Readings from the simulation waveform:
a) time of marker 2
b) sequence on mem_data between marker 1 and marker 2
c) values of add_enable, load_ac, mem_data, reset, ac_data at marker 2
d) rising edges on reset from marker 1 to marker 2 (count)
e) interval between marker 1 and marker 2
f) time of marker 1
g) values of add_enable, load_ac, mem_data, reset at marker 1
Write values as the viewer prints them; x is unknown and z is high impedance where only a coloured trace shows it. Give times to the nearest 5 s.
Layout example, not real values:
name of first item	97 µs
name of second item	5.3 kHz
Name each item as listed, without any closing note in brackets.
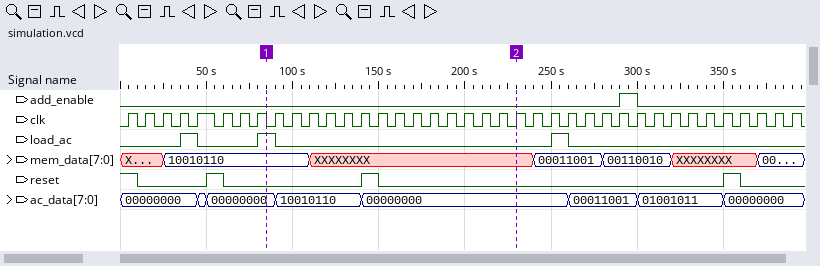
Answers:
time of marker 2	230 s
sequence on mem_data between marker 1 and marker 2	10010110, XXXXXXXX
values of add_enable, load_ac, mem_data, reset, ac_data at marker 2	add_enable=0, load_ac=0, mem_data=XXXXXXXX, reset=0, ac_data=00000000
rising edges on reset from marker 1 to marker 2	1
interval between marker 1 and marker 2	145 s
time of marker 1	85 s
values of add_enable, load_ac, mem_data, reset at marker 1	add_enable=0, load_ac=1, mem_data=10010110, reset=0
